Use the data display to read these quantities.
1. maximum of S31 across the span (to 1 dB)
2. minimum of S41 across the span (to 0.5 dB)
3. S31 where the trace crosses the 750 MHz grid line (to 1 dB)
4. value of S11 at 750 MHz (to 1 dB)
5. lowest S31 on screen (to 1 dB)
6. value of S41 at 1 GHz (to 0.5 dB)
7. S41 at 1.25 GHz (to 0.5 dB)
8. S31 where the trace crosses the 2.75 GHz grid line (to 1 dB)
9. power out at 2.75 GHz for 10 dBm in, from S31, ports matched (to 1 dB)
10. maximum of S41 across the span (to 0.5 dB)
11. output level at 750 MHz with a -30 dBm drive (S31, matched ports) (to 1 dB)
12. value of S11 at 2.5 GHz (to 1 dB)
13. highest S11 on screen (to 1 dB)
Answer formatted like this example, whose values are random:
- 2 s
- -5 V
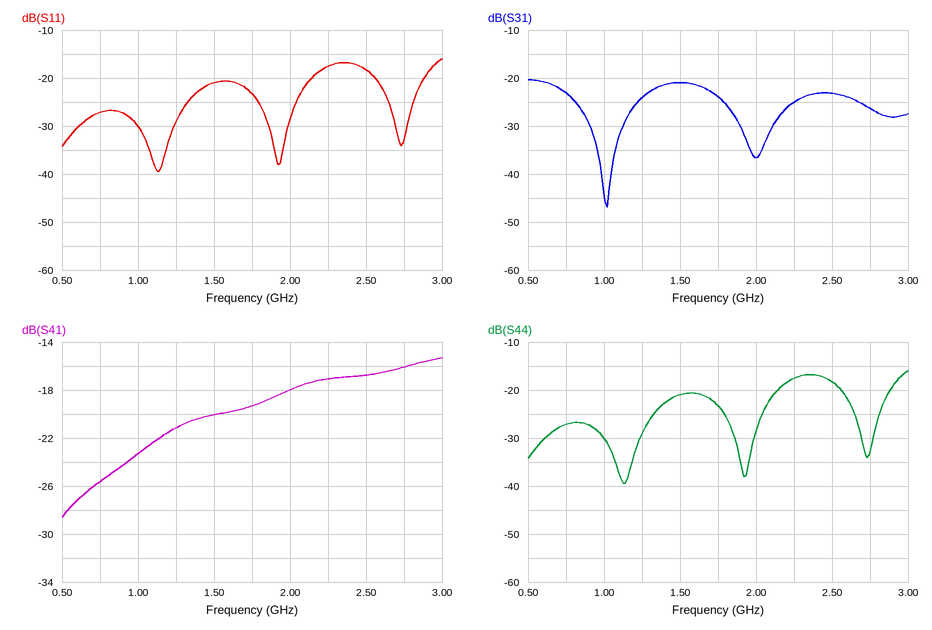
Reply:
- -20 dB
- -28.5 dB
- -23 dB
- -27 dB
- -47 dB
- -23.5 dB
- -21.0 dB
- -26 dB
- -16 dBm
- -15.5 dB
- -53 dBm
- -18 dB
- -16 dB
